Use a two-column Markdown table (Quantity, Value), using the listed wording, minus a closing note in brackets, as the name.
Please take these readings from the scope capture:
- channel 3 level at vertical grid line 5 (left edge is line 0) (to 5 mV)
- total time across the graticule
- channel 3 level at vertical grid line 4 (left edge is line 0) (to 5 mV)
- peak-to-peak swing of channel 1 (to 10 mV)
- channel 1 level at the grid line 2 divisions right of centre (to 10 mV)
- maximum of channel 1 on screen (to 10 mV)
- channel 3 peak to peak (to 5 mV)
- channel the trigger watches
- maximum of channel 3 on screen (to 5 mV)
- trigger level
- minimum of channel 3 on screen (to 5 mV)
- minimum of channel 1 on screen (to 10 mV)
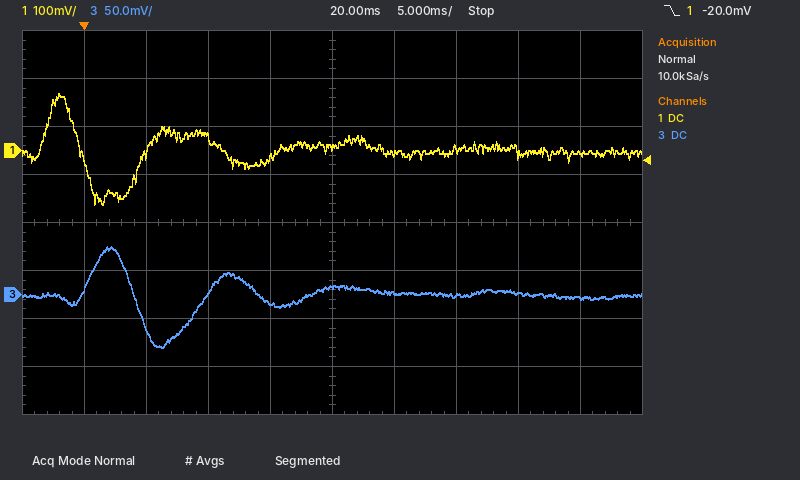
| Quantity | Value |
|---|---|
| channel 3 level at vertical grid line 5 (left edge is line 0) | 10 mV |
| total time across the graticule | 50 ms |
| channel 3 level at vertical grid line 4 (left edge is line 0) | -10 mV |
| peak-to-peak swing of channel 1 | 230 mV |
| channel 1 level at the grid line 2 divisions right of centre | 0 mV |
| maximum of channel 1 on screen | 120 mV |
| channel 3 peak to peak | 105 mV |
| channel the trigger watches | channel 1 |
| maximum of channel 3 on screen | 50 mV |
| trigger level | -20.0 mV |
| minimum of channel 3 on screen | -55 mV |
| minimum of channel 1 on screen | -110 mV |
